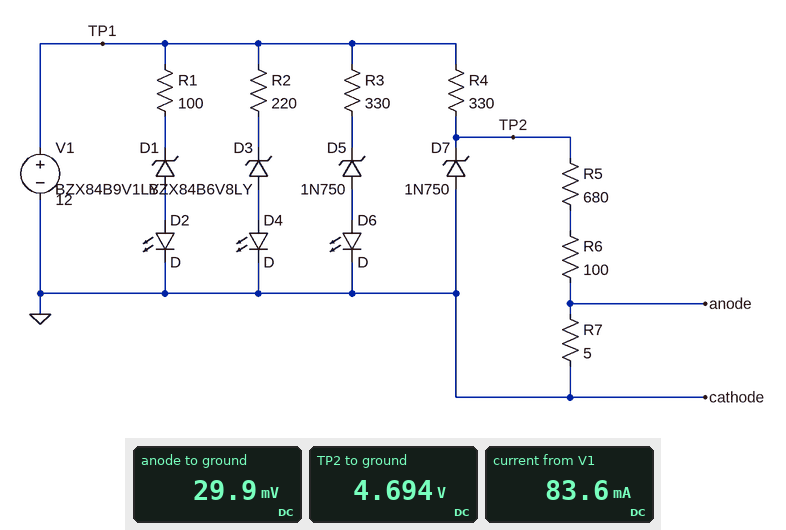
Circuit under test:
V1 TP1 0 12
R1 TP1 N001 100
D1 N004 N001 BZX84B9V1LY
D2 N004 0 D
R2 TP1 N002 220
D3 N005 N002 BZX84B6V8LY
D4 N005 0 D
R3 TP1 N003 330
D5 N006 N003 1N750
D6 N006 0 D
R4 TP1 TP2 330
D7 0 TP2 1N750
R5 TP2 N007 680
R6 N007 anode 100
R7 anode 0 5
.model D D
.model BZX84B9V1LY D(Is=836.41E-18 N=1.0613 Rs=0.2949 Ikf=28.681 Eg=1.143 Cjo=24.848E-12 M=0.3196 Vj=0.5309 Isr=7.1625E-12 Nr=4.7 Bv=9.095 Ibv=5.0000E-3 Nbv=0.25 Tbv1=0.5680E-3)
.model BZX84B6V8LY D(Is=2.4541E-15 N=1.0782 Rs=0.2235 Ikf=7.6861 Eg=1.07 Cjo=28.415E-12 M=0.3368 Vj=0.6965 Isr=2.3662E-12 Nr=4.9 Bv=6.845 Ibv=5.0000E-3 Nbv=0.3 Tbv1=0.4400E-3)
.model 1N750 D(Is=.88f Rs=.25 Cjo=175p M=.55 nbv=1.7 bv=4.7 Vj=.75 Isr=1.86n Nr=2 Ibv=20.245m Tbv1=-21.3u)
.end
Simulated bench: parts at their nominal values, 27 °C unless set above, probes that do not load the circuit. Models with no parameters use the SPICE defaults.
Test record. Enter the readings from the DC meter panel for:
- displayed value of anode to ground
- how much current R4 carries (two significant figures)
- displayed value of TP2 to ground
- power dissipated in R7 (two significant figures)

29.9 mV
22 mA
4.694 V
180 µW
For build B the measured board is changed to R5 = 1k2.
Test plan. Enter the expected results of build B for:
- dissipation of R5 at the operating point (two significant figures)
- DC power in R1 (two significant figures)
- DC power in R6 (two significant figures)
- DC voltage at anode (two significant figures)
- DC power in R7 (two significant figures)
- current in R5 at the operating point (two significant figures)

16 mW
46 mW
1.3 mW
18 mV
65 µW
3.6 mA
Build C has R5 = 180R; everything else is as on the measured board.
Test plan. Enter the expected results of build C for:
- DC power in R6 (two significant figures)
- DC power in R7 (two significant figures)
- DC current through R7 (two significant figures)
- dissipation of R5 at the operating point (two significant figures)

27 mW
1.3 mW
16 mA
48 mW
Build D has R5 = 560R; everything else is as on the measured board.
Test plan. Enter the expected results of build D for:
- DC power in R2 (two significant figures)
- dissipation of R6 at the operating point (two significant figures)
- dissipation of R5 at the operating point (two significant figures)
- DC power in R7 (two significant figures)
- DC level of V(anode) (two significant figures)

88 mW
5.0 mW
28 mW
250 µW
35 mV
